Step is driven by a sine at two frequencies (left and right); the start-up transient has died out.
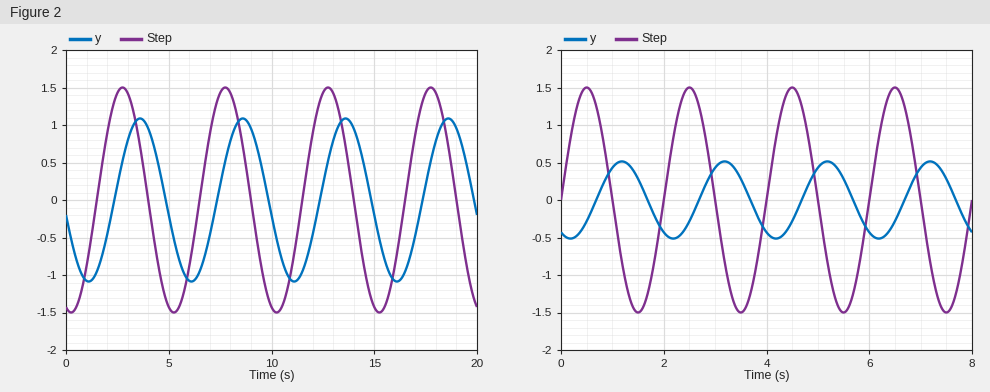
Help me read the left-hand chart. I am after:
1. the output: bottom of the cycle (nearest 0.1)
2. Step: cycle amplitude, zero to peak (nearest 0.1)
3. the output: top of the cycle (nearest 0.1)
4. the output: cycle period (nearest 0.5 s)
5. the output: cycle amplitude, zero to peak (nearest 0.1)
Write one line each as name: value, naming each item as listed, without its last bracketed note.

the output: bottom of the cycle: -1.1
Step: cycle amplitude, zero to peak: 1.5
the output: top of the cycle: 1.1
the output: cycle period: 5.0 s
the output: cycle amplitude, zero to peak: 1.1
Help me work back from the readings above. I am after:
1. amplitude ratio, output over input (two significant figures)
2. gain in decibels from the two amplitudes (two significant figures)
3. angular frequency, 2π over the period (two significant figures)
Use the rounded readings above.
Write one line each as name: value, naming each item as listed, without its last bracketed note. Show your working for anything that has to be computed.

amplitude ratio, output over input: 1.1 / 1.5 = 0.73
gain in decibels from the two amplitudes: 20 log10(1.1 / 1.5) = -2.7 dB
angular frequency, 2π over the period: 2π / 5 = 1.3 rad/s
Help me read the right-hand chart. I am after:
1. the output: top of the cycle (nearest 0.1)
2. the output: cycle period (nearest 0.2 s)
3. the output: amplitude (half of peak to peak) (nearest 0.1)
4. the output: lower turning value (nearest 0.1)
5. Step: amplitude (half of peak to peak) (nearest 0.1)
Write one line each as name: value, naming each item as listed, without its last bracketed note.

the output: top of the cycle: 0.5
the output: cycle period: 2.0 s
the output: amplitude (half of peak to peak): 0.5
the output: lower turning value: -0.5
Step: amplitude (half of peak to peak): 1.5
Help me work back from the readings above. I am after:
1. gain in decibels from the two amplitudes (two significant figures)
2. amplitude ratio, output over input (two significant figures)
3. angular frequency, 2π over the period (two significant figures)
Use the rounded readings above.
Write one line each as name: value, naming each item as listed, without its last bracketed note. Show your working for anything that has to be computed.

gain in decibels from the two amplitudes: 20 log10(0.5 / 1.5) = -9.5 dB
amplitude ratio, output over input: 0.5 / 1.5 = 0.33
angular frequency, 2π over the period: 2π / 2 = 3.1 rad/s
